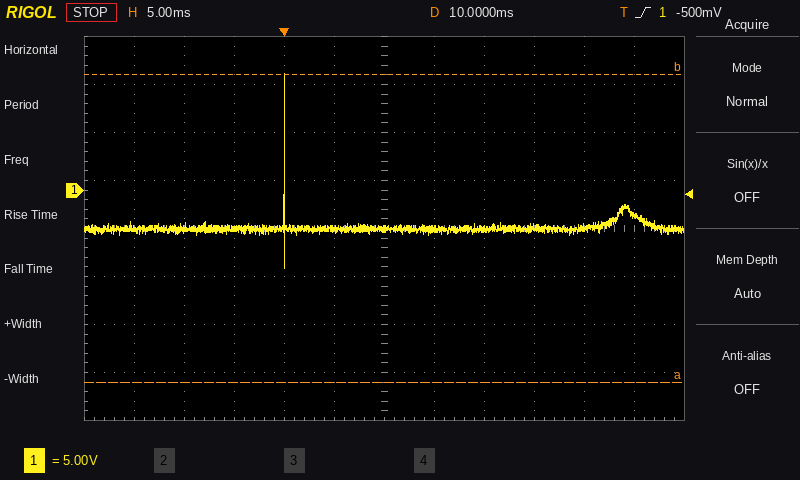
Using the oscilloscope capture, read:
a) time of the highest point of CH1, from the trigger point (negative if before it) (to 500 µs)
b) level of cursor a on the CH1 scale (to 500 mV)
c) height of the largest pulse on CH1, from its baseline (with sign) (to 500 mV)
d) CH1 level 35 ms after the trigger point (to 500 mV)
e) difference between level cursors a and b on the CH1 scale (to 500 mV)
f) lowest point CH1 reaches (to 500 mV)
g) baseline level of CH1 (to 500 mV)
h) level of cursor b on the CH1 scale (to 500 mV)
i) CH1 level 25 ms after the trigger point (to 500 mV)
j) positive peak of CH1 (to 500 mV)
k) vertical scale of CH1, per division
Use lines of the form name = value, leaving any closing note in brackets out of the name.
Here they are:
time of the highest point of CH1, from the trigger point (negative if before it) = 0.0 ms
level of cursor a on the CH1 scale = -20.0 V
height of the largest pulse on CH1, from its baseline (with sign) = +16.0 V
CH1 level 35 ms after the trigger point = -2.5 V
difference between level cursors a and b on the CH1 scale = 32.0 V
lowest point CH1 reaches = -8.0 V
baseline level of CH1 = -4.0 V
level of cursor b on the CH1 scale = 12.0 V
CH1 level 25 ms after the trigger point = -4.0 V
positive peak of CH1 = 12.0 V
vertical scale of CH1, per division = 5 V
